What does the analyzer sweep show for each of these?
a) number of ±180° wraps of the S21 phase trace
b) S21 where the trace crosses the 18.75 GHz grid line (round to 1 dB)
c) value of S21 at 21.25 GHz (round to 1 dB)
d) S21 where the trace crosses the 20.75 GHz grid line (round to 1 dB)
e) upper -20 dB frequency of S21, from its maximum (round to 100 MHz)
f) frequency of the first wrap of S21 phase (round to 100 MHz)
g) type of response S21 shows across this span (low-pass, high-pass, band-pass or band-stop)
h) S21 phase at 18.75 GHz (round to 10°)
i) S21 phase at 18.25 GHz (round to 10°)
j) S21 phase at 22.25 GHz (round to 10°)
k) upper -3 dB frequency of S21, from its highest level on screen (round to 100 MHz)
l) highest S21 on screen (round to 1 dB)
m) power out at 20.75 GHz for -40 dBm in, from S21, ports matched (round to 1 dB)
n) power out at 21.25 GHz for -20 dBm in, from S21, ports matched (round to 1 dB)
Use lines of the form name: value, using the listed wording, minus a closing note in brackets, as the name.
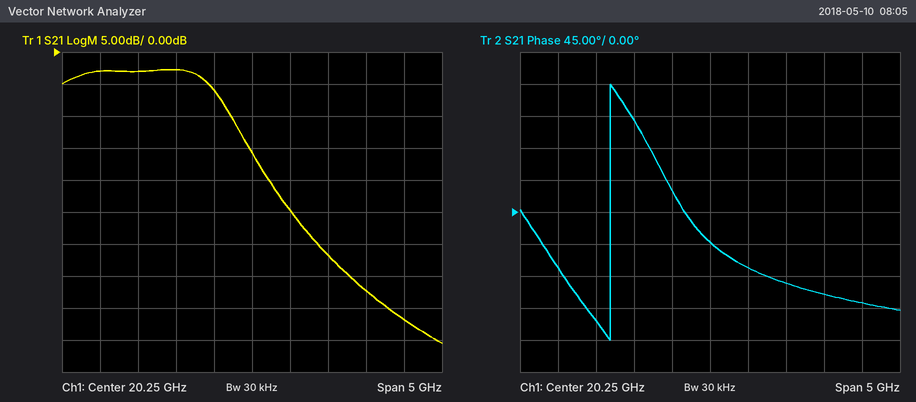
number of ±180° wraps of the S21 phase trace: 1
S21 where the trace crosses the 18.75 GHz grid line: -3 dB
value of S21 at 21.25 GHz: -32 dB
S21 where the trace crosses the 20.75 GHz grid line: -25 dB
upper -20 dB frequency of S21, from its maximum: 20.6 GHz
frequency of the first wrap of S21 phase: 18.9 GHz
type of response S21 shows across this span: low-pass
S21 phase at 18.75 GHz: -150°
S21 phase at 18.25 GHz: -80°
S21 phase at 22.25 GHz: -130°
upper -3 dB frequency of S21, from its highest level on screen: 19.7 GHz
highest S21 on screen: -3 dB
power out at 20.75 GHz for -40 dBm in, from S21, ports matched: -65 dBm
power out at 21.25 GHz for -20 dBm in, from S21, ports matched: -52 dBm
